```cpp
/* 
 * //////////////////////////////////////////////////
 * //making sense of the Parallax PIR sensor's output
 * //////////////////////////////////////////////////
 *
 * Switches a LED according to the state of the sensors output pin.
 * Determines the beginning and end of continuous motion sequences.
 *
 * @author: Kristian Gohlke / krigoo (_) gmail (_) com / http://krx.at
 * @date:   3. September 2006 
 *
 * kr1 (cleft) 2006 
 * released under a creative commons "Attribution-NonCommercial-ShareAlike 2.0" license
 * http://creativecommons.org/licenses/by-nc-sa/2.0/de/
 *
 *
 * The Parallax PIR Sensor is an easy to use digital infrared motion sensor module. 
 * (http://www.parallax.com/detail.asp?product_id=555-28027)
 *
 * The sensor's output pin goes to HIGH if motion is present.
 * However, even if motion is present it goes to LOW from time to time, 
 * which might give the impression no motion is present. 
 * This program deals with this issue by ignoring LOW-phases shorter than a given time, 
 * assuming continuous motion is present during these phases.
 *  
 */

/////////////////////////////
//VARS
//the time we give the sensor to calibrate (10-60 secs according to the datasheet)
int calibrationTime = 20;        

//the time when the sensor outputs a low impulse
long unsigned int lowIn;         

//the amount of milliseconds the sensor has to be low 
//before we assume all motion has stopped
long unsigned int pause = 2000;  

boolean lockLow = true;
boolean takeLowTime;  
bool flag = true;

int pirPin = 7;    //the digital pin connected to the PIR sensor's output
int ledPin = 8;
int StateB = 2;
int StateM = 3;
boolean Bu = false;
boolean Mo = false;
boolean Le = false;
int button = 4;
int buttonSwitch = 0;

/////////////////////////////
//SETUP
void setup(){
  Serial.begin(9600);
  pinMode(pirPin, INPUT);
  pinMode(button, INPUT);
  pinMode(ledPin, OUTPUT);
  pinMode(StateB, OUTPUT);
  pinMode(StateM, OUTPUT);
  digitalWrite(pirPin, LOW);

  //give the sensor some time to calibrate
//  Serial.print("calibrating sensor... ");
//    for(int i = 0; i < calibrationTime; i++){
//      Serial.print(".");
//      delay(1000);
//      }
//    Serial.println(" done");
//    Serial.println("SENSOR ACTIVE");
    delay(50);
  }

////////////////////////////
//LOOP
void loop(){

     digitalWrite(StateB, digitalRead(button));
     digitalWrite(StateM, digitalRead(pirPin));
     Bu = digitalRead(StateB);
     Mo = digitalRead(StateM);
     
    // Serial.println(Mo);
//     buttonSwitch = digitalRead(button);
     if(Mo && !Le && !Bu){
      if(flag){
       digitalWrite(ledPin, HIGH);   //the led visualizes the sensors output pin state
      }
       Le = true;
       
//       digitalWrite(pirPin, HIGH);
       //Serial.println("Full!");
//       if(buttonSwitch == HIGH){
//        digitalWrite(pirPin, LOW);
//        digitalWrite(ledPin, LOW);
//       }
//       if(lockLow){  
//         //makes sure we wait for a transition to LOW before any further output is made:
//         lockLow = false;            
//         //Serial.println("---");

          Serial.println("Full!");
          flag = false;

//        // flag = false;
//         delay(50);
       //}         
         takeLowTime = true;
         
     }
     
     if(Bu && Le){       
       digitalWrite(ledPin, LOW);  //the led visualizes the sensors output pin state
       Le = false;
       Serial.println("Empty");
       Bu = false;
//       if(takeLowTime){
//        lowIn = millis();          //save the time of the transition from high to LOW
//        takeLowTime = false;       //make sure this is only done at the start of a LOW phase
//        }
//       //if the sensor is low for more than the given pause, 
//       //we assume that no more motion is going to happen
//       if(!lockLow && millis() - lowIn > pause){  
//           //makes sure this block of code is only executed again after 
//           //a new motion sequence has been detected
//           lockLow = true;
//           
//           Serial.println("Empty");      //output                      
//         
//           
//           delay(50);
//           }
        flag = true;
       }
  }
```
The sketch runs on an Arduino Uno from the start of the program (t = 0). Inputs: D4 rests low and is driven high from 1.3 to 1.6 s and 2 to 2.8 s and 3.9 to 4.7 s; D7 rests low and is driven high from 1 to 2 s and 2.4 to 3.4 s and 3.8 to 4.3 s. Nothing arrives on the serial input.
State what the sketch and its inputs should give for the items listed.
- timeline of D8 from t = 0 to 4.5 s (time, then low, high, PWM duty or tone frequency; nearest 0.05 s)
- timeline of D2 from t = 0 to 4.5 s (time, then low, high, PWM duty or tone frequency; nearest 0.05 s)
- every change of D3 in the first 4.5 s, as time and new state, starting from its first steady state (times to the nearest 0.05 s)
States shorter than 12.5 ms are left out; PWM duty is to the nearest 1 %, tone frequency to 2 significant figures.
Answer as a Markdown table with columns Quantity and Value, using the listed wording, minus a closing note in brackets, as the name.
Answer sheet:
| Quantity | Value |
|---|---|
| timeline of D8 from t = 0 to 4.5 s | 0 s low; 1 s high; 1.3 s low; 1.6 s high; 2 s low; 2.8 s high; 3.9 s low |
| timeline of D2 from t = 0 to 4.5 s | 0 s low; 1.3 s high; 1.6 s low; 2 s high; 2.8 s low; 3.9 s high |
| every change of D3 in the first 4.5 s, as time and new state, starting from its first steady state | 0 s low; 1 s high; 2 s low; 2.4 s high; 3.4 s low; 3.8 s high; 4.3 s low |
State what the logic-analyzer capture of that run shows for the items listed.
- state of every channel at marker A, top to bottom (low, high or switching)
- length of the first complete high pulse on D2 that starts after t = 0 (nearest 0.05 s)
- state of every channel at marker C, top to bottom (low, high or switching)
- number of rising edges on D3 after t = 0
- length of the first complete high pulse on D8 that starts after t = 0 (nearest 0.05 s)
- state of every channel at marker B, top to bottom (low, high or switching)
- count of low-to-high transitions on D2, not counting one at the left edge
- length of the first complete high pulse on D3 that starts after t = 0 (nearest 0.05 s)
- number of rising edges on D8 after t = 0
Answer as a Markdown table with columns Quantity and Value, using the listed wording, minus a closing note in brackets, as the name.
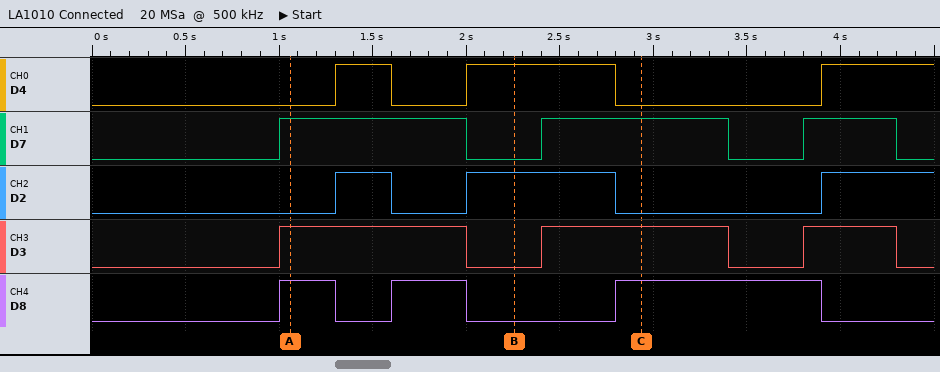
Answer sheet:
| Quantity | Value |
|---|---|
| state of every channel at marker A, top to bottom | D4 low, D7 high, D2 low, D3 high, D8 high |
| length of the first complete high pulse on D2 that starts after t = 0 | 0.30 s |
| state of every channel at marker C, top to bottom | D4 low, D7 high, D2 low, D3 high, D8 high |
| number of rising edges on D3 after t = 0 | 3 |
| length of the first complete high pulse on D8 that starts after t = 0 | 0.30 s |
| state of every channel at marker B, top to bottom | D4 high, D7 low, D2 high, D3 low, D8 low |
| count of low-to-high transitions on D2, not counting one at the left edge | 3 |
| length of the first complete high pulse on D3 that starts after t = 0 | 1.00 s |
| number of rising edges on D8 after t = 0 | 3 |
